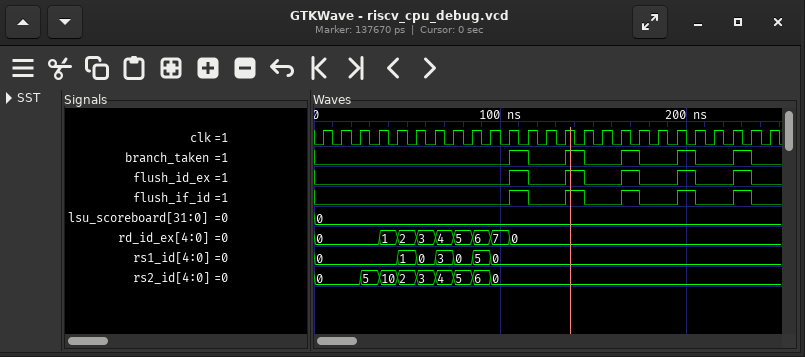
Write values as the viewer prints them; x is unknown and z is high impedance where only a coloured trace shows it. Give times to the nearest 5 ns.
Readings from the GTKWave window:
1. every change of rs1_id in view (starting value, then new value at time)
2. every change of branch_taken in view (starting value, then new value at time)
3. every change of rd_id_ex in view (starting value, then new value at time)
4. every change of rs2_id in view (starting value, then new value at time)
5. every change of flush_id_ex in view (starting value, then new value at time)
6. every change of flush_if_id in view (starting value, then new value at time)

0, 1 at 45 ns, 0 at 55 ns, 3 at 65 ns, 0 at 75 ns, 5 at 85 ns, 0 at 95 ns
0, 1 at 105 ns, 0 at 115 ns, 1 at 135 ns, 0 at 145 ns, 1 at 165 ns, 0 at 175 ns, 1 at 195 ns, 0 at 205 ns, 1 at 225 ns, 0 at 235 ns
0, 1 at 35 ns, 2 at 45 ns, 3 at 55 ns, 4 at 65 ns, 5 at 75 ns, 6 at 85 ns, 7 at 95 ns, 0 at 105 ns
0, 5 at 25 ns, 10 at 35 ns, 2 at 45 ns, 3 at 55 ns, 4 at 65 ns, 5 at 75 ns, 6 at 85 ns, 0 at 95 ns
0, 1 at 105 ns, 0 at 115 ns, 1 at 135 ns, 0 at 145 ns, 1 at 165 ns, 0 at 175 ns, 1 at 195 ns, 0 at 205 ns, 1 at 225 ns, 0 at 235 ns
0, 1 at 105 ns, 0 at 115 ns, 1 at 135 ns, 0 at 145 ns, 1 at 165 ns, 0 at 175 ns, 1 at 195 ns, 0 at 205 ns, 1 at 225 ns, 0 at 235 ns
